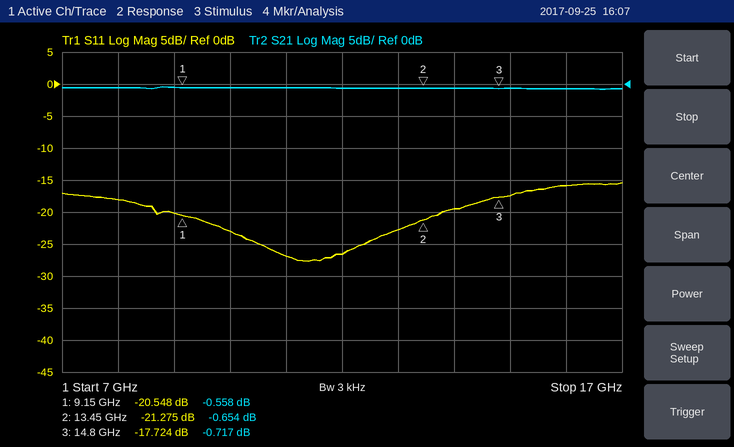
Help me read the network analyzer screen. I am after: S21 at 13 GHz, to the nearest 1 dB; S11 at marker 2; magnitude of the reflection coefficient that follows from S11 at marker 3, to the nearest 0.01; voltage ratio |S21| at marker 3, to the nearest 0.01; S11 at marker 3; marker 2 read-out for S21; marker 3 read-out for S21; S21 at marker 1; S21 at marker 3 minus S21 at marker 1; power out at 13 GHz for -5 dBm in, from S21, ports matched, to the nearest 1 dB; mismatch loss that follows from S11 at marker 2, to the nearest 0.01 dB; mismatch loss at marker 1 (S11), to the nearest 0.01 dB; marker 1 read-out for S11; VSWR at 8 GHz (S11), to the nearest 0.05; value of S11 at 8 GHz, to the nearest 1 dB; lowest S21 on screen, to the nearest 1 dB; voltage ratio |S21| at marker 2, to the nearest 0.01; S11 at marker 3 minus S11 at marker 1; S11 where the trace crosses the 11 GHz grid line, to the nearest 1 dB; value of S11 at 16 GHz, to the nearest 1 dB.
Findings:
-1 dB
-21.275 dB
0.13
0.92
-17.724 dB
-0.654 dB
-0.717 dB
-0.558 dB
-0.159 dB
-6 dBm
0.03 dB
0.04 dB
-20.548 dB
1.30
-18 dB
-1 dB
0.93
2.824 dB
-27 dB
-16 dB
